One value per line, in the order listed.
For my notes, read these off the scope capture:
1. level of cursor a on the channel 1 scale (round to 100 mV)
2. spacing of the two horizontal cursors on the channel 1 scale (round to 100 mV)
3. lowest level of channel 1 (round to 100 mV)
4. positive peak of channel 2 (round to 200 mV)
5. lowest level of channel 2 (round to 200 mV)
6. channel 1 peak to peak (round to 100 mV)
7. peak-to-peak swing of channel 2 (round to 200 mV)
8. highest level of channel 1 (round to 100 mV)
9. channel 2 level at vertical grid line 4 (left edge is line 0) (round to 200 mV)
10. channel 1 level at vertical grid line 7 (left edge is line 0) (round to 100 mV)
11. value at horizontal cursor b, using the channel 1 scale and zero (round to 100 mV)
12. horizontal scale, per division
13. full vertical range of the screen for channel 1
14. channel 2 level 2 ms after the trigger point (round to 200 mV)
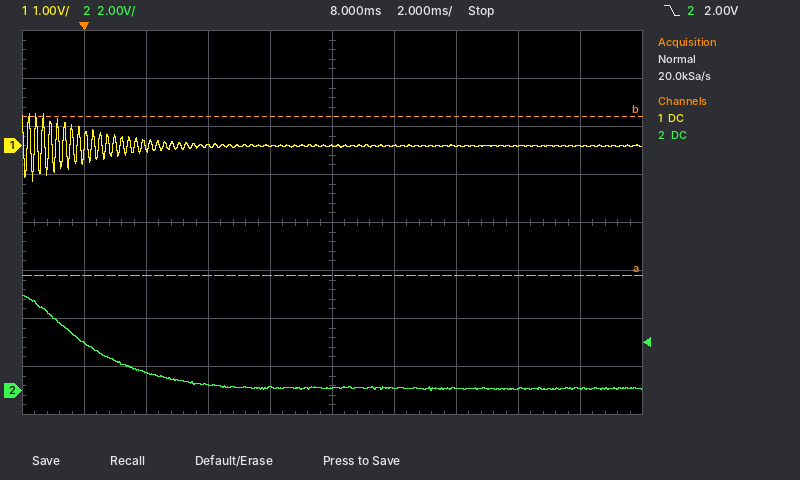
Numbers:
-2.7 V
3.3 V
-700 mV
4.0 V
0.0 V
1.4 V
4.0 V
700 mV
200 mV
0.0 V
600 mV
2 ms
8 V
800 mV
